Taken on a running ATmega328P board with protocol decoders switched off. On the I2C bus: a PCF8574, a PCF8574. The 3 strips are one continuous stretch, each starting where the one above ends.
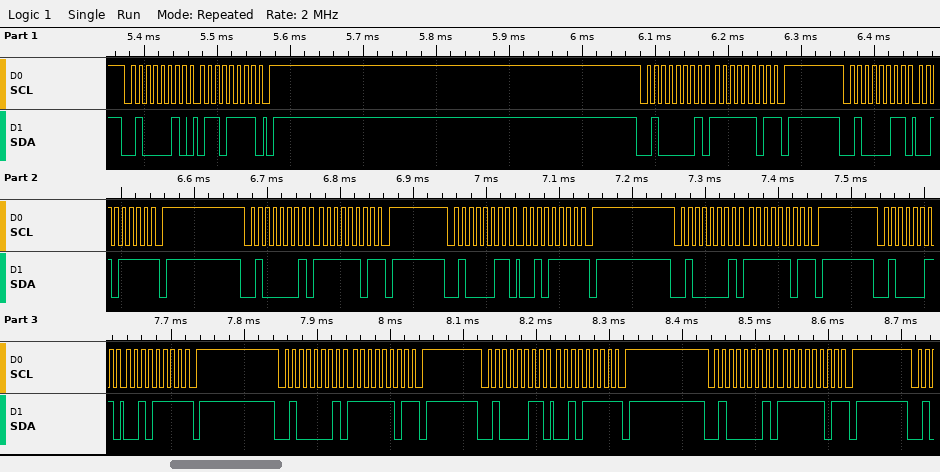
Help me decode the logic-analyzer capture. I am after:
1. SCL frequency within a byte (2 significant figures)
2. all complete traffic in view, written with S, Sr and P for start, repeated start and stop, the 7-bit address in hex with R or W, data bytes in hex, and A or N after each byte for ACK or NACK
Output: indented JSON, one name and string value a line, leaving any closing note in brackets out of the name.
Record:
{
  "SCL frequency within a byte": "100 kHz",
  "all complete traffic in view, written with S, Sr and P for start, repeated start and stop, the 7-bit address in hex with R or W, data bytes in hex, and A or N after each byte for ACK or NACK": "S 21W A 6F A P S 20R A FD N P S 21R A 2F N P S 20R A FD N P S 21R A 2F N P S 20R A FD N P S 21R A 2F N P S 20R A FD N P S 21R A 2F N P S 20R A FD N P"
}
